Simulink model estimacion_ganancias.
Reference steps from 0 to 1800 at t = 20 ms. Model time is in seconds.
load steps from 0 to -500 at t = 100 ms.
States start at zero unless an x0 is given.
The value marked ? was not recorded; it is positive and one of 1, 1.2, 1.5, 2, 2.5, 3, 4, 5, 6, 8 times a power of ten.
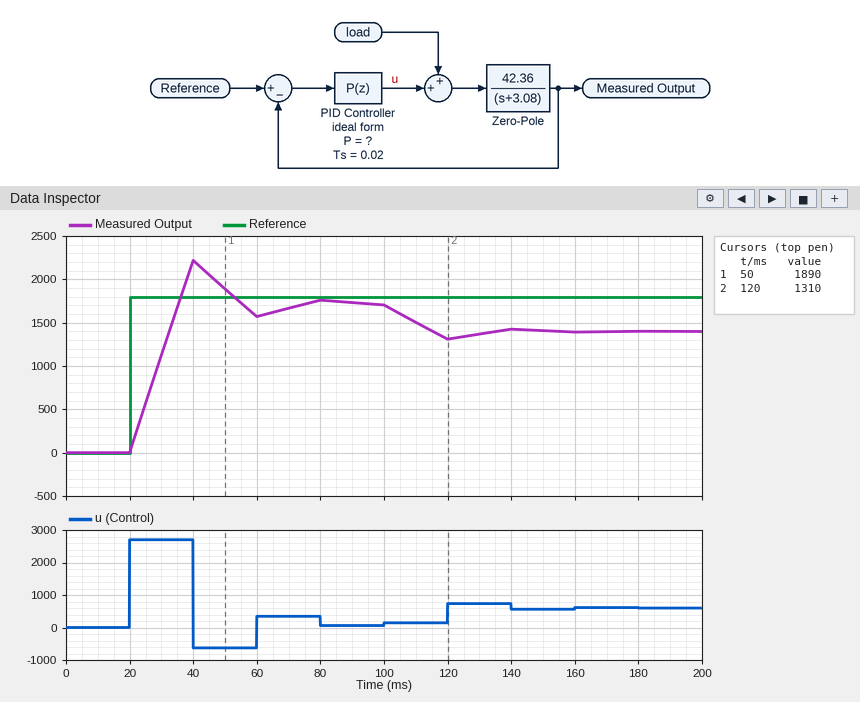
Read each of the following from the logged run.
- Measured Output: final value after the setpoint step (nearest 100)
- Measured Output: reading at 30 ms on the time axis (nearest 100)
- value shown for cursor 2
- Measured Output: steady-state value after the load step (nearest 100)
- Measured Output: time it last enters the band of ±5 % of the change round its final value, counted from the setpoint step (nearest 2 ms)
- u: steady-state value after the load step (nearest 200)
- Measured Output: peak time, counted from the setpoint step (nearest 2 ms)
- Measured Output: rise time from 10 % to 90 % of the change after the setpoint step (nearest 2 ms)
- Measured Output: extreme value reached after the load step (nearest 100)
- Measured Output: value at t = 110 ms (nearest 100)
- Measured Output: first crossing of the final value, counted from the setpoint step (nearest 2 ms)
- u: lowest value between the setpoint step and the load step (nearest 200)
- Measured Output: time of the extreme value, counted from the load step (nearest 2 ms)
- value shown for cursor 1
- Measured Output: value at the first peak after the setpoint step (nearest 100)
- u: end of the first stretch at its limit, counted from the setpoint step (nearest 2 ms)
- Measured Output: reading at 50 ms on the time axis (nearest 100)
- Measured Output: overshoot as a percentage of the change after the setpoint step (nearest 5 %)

1700
1100
1310
1400
46 ms
600
20 ms
12 ms
1300
1500
16 ms
-600
20 ms
1890
2200
20 ms
1900
30 %
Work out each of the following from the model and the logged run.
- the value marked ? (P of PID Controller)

1.5
